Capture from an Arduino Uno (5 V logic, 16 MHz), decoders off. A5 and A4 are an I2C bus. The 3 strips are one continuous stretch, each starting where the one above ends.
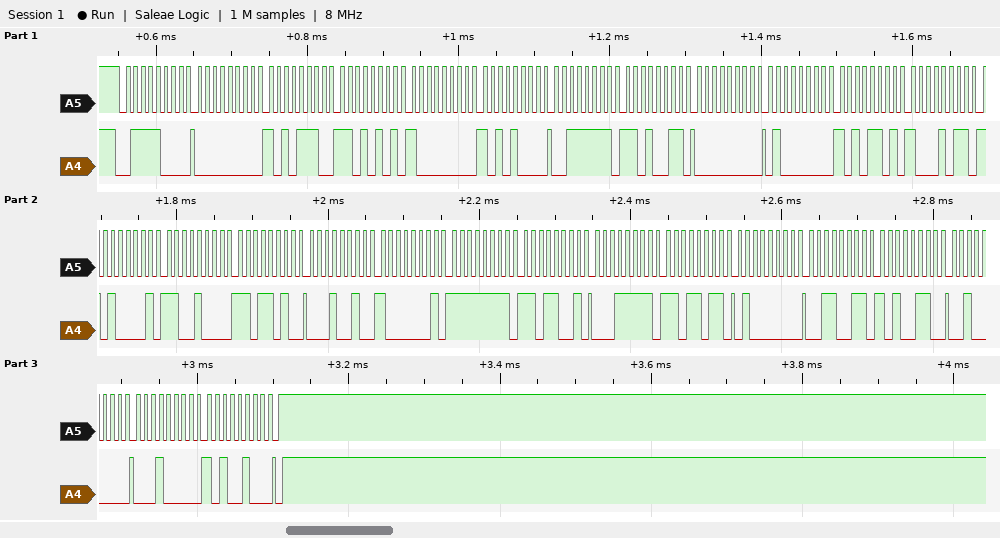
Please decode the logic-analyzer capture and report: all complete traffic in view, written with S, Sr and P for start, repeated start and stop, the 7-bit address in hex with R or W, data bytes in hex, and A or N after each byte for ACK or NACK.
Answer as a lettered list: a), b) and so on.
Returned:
a) S 3CW A 00 A AE A D5 A 80 A A8 A 3F A D3 A 00 A 40 A AD A 8B A A1 A C8 A DA A 12 A 81 A FF A D9 A 1F A DB A 40 A 33 A A6 A 20 A 10 A A4 A P
